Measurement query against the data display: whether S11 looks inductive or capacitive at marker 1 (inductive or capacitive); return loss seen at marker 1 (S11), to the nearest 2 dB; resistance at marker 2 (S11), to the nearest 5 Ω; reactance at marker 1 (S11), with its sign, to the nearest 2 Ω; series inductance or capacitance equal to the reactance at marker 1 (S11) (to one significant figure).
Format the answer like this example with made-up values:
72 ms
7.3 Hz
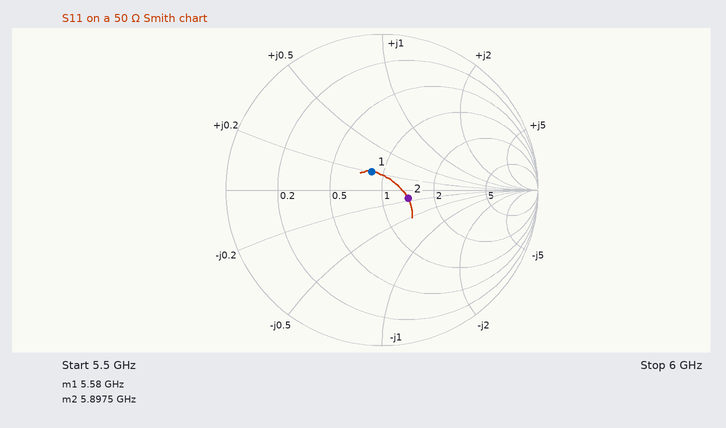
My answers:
inductive
18 dB
70 Ω
+10 Ω
300 pH
